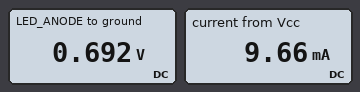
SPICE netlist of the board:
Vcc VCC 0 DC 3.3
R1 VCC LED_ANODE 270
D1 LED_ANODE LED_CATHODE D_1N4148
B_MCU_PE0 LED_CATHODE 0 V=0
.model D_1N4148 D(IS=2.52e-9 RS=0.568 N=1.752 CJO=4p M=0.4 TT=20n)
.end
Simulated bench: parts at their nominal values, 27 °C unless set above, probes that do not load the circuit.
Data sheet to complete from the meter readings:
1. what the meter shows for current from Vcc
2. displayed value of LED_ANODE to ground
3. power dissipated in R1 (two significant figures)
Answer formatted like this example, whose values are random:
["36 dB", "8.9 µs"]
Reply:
["9.66 mA", "0.692 V", "25 mW"]
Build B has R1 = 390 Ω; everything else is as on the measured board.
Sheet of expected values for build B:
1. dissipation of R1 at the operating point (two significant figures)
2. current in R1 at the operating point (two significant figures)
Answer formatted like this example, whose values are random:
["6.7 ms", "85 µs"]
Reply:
["18 mW", "6.7 mA"]
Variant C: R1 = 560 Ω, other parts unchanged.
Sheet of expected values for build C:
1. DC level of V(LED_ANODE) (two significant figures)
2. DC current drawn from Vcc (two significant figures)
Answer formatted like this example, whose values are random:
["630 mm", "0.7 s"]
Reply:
["660 mV", "4.7 mA"]
